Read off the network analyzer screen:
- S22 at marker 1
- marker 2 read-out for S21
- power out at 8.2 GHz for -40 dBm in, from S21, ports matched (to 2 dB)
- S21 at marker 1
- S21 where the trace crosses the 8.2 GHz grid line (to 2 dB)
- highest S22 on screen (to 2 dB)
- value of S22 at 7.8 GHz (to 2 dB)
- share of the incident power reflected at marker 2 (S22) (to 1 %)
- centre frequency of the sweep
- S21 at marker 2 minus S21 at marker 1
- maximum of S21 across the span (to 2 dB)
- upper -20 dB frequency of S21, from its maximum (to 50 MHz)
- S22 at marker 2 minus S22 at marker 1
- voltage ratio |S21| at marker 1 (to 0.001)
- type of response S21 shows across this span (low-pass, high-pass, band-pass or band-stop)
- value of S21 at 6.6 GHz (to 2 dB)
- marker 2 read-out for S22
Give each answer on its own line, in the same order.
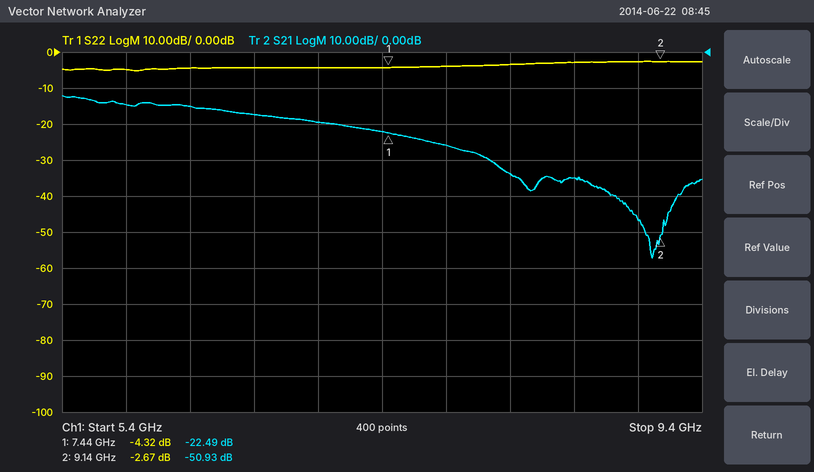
-4.32 dB
-50.93 dB
-74 dBm
-22.49 dB
-34 dB
-2 dB
-4 dB
54 %
7.4 GHz
-28.44 dB
-12 dB
8.15 GHz
1.65 dB
0.075
low-pass
-18 dB
-2.67 dB
